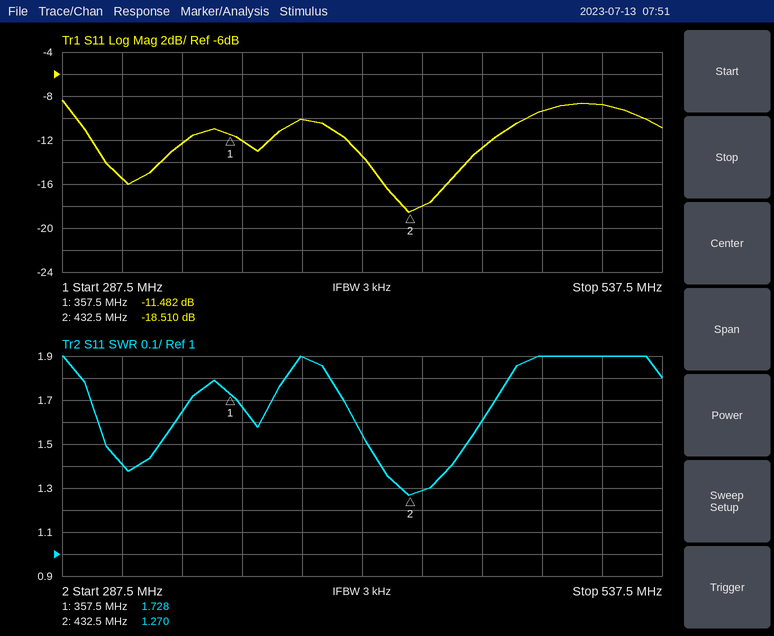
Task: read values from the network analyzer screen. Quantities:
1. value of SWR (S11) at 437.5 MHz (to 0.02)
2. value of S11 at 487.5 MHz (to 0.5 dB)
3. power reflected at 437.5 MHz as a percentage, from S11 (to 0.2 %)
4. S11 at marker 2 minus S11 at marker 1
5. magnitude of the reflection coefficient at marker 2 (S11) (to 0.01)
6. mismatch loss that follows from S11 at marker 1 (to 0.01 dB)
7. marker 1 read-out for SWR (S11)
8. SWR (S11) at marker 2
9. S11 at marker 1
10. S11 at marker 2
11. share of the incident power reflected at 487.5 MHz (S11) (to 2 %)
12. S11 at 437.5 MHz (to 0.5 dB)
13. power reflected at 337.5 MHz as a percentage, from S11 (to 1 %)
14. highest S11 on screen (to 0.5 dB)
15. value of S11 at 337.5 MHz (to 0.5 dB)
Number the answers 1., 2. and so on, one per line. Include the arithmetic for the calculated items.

1. 1.28
2. -9.5 dB
3. 10^(-18/10) ≈ 1.6 %
4. -18.51 − (-11.482) = -7.028 dB
5. 10^(-18.51/20) ≈ 0.12
6. −10 log10(1 − 10^(-11.482/10)) ≈ 0.32 dB
7. 1.728
8. 1.270
9. -11.482 dB
10. -18.510 dB
11. 10^(-9.5/10) ≈ 11.2 %, so 12 % to the nearest 2 %
12. -18.0 dB
13. 10^(-12.5/10) ≈ 6 %
14. -8.5 dB
15. -12.5 dB
